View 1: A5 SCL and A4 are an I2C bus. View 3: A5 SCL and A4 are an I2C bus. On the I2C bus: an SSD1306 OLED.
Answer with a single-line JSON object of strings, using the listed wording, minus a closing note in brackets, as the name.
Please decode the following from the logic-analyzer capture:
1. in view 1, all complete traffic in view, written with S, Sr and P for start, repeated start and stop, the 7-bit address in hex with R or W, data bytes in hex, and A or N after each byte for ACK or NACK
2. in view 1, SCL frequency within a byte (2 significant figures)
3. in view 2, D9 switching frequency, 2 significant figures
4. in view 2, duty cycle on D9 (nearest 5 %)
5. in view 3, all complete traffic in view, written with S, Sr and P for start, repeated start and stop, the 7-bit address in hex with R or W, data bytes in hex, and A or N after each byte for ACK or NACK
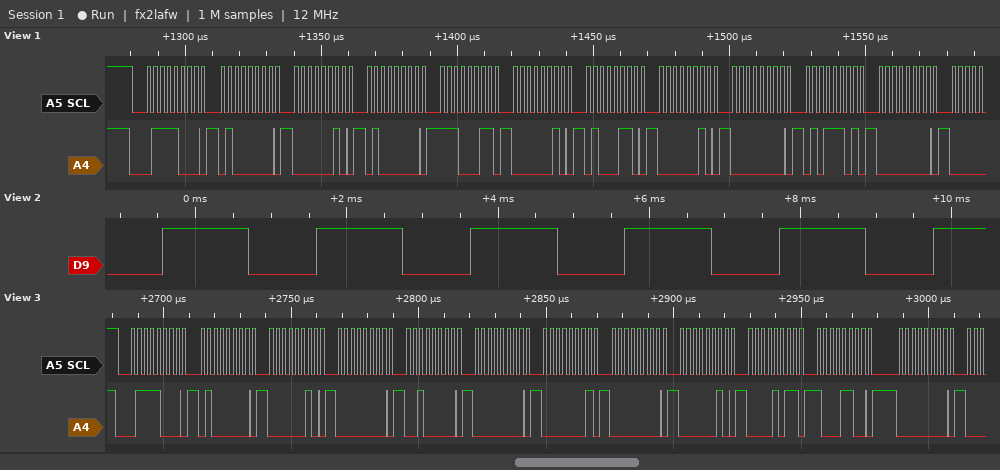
{"in view 1, all complete traffic in view, written with S, Sr and P for start, repeated start and stop, the 7-bit address in hex with R or W, data bytes in hex, and A or N after each byte for ACK or NACK": "S 3CW A 40 A 02 A 40 A E3 A 02 A 46 A 02 A 00 A 5D A 00 A", "in view 1, SCL frequency within a byte": "400 kHz", "in view 2, D9 switching frequency, 2 significant figures": "490 Hz", "in view 2, duty cycle on D9": "55 %", "in view 3, all complete traffic in view, written with S, Sr and P for start, repeated start and stop, the 7-bit address in hex with R or W, data bytes in hex, and A or N after each byte for ACK or NACK": "S 3CW A 40 A 02 A 00 A 20 A 00 A 01 A 00 A 02 A 0B A 8C A 00 A"}
